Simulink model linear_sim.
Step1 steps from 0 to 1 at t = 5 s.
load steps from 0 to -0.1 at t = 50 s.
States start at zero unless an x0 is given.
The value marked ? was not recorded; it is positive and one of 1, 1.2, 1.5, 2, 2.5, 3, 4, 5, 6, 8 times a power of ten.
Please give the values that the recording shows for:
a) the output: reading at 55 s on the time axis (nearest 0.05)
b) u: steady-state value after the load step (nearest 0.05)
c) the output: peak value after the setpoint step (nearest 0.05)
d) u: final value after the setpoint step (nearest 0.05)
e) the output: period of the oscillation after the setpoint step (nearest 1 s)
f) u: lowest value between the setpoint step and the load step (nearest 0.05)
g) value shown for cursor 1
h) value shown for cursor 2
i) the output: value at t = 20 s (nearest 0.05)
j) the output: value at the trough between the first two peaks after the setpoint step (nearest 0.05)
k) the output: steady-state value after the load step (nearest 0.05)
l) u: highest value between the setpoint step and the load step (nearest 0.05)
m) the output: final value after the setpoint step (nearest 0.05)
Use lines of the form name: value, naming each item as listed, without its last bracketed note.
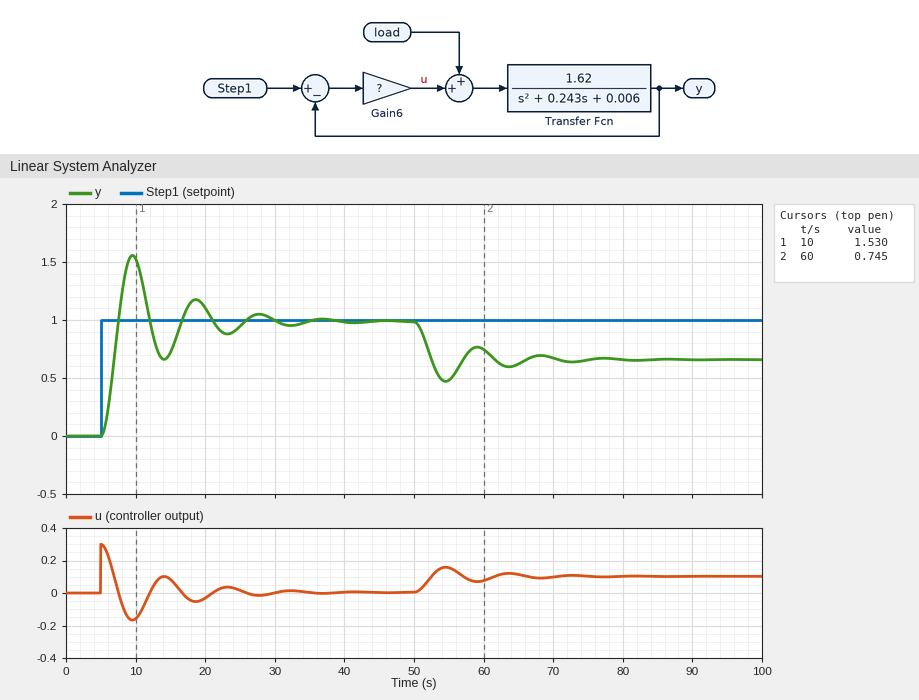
the output: reading at 55 s on the time axis: 0.50
u: steady-state value after the load step: 0.10
the output: peak value after the setpoint step: 1.55
u: final value after the setpoint step: 0.00
the output: period of the oscillation after the setpoint step: 9 s
u: lowest value between the setpoint step and the load step: -0.15
value shown for cursor 1: 1.530
value shown for cursor 2: 0.745
the output: value at t = 20 s: 1.10
the output: value at the trough between the first two peaks after the setpoint step: 0.65
the output: steady-state value after the load step: 0.65
u: highest value between the setpoint step and the load step: 0.30
the output: final value after the setpoint step: 1.00
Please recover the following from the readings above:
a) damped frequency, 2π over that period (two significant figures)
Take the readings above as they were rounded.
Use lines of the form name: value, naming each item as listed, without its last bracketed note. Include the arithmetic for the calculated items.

damped frequency, 2π over that period: 2π / 9 = 0.70 rad/s
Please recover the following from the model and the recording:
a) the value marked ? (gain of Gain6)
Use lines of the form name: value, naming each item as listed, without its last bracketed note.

the value marked ?: 0.3
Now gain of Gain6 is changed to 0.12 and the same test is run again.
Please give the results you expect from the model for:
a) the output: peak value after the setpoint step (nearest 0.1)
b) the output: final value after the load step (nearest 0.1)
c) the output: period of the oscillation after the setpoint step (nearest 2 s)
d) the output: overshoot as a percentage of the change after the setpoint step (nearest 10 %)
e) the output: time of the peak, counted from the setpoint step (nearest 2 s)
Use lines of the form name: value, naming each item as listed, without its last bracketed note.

the output: peak value after the setpoint step: 1.4
the output: final value after the load step: 0.2
the output: period of the oscillation after the setpoint step: 14 s
the output: overshoot as a percentage of the change after the setpoint step: 40 %
the output: time of the peak, counted from the setpoint step: 8 s
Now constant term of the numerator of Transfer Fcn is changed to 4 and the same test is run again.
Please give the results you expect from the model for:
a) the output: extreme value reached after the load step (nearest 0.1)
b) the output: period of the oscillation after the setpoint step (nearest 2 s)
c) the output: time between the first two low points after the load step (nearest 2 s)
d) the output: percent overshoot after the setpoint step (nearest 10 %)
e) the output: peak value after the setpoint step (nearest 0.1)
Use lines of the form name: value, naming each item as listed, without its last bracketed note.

the output: extreme value reached after the load step: 0.4
the output: period of the oscillation after the setpoint step: 6 s
the output: time between the first two low points after the load step: 6 s
the output: percent overshoot after the setpoint step: 70 %
the output: peak value after the setpoint step: 1.7
